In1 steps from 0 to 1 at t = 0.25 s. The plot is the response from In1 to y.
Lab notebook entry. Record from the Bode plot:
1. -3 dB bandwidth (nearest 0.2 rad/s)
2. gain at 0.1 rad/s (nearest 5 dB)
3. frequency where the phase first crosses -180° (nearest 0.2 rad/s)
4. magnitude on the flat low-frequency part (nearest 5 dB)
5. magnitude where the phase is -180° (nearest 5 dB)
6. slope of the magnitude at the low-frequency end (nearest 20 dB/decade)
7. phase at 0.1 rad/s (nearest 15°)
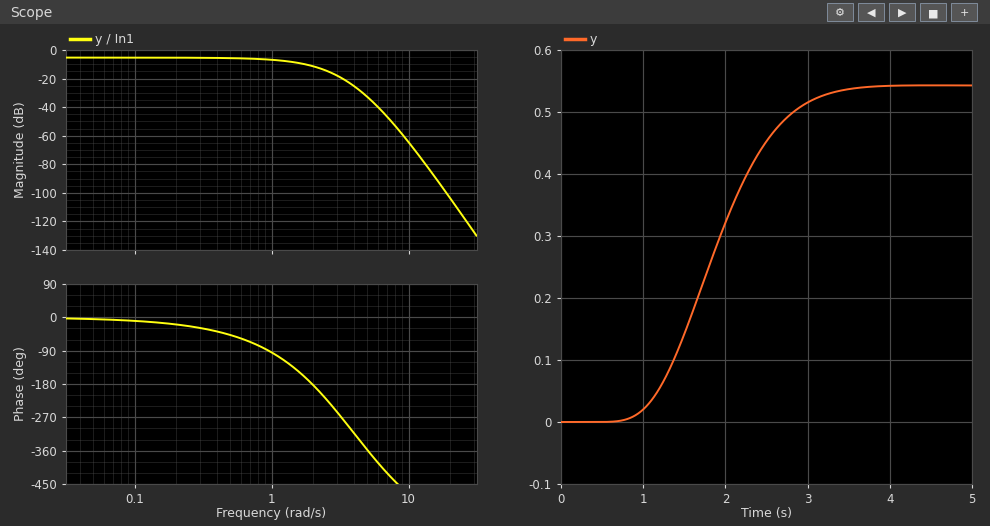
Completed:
1.4 rad/s
-5 dB
2.0 rad/s
-5 dB
-10 dB
0 dB/decade
-15°
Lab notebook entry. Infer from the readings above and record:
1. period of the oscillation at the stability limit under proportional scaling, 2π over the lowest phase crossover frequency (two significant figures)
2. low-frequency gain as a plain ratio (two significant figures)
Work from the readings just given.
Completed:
3.1 s
0.56
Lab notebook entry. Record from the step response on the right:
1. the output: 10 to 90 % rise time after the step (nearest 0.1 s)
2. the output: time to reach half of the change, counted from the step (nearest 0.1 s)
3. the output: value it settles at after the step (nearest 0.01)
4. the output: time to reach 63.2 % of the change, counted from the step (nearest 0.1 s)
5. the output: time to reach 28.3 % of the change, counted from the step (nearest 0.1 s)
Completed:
1.5 s
1.6 s
0.54
1.8 s
1.3 s
